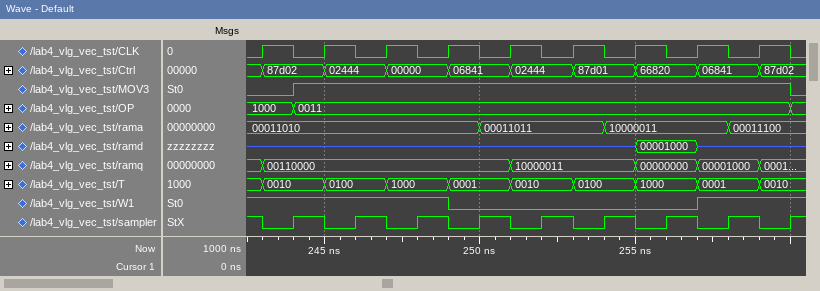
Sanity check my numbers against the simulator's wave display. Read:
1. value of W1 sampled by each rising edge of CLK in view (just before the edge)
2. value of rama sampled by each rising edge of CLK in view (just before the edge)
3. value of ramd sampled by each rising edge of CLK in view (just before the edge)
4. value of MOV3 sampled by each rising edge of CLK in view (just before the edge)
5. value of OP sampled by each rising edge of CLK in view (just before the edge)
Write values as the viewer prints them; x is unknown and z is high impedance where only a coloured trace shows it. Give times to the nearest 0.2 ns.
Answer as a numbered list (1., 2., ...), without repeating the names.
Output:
1. 1 1 1 1 0 0 0 0 1
2. 00011010, 00011010, 00011010, 00011010, 00011011, 00011011, 10000011, 10000011, 00011100
3. z, z, z, z, z, z, z, 00001000, z
4. 0 1 1 1 1 1 1 1 1
5. 1000, 0011, 0011, 0011, 0011, 0011, 0011, 0011, 0011
